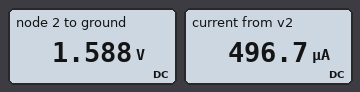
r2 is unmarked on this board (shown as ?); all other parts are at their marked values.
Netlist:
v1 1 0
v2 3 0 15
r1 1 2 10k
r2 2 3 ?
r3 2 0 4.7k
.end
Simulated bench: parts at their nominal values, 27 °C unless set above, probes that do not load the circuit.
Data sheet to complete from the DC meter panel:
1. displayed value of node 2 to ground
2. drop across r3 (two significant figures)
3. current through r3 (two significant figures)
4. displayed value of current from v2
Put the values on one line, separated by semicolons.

1.588 V; 1.6 V; 340 µA; 496.7 µA
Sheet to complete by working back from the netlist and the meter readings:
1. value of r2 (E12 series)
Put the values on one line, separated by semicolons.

27 kΩ
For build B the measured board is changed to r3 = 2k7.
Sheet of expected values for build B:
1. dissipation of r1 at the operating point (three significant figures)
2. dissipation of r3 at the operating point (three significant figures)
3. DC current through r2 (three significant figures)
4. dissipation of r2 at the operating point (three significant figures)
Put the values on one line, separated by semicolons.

120 µW; 444 µW; 515 µA; 7.16 mW
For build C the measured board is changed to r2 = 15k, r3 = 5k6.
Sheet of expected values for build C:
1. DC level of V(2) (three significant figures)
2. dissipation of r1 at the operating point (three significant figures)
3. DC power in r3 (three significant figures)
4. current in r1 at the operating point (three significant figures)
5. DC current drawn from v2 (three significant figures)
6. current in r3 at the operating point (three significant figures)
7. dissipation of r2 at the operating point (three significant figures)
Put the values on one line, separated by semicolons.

2.90 V; 839 µW; 1.50 mW; 290 µA; 807 µA; 517 µA; 9.77 mW
